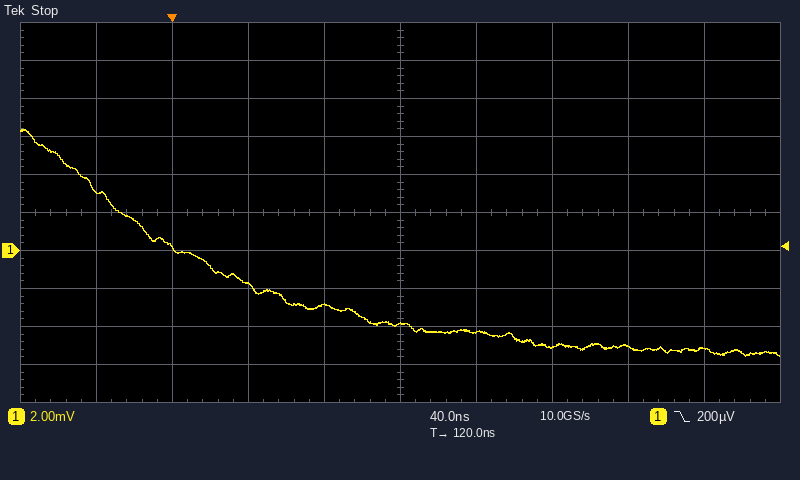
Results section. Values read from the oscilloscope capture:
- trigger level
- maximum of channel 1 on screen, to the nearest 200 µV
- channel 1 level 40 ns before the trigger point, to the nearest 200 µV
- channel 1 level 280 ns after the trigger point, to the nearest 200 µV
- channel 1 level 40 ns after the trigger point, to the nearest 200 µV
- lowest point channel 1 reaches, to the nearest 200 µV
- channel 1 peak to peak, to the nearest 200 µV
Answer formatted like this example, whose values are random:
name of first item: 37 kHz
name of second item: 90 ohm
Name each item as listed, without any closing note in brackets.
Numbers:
trigger level: 200 µV
maximum of channel 1 on screen, to the nearest 200 µV: 6.4 mV
channel 1 level 40 ns before the trigger point, to the nearest 200 µV: 3.2 mV
channel 1 level 280 ns after the trigger point, to the nearest 200 µV: -5.2 mV
channel 1 level 40 ns after the trigger point, to the nearest 200 µV: -1.8 mV
lowest point channel 1 reaches, to the nearest 200 µV: -5.6 mV
channel 1 peak to peak, to the nearest 200 µV: 12.0 mV
